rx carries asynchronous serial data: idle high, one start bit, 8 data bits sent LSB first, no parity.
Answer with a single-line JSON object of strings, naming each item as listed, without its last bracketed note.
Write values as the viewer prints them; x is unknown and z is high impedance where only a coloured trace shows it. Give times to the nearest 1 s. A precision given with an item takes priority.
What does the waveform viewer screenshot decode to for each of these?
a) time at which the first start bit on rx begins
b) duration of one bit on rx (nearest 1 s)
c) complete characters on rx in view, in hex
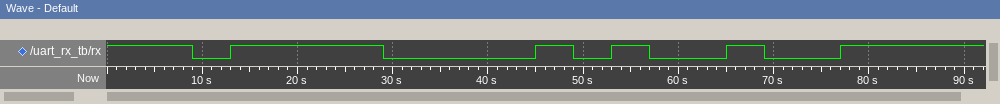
{"time at which the first start bit on rx begins": "9 s", "duration of one bit on rx": "4 s", "complete characters on rx in view, in hex": "0F, C9"}
